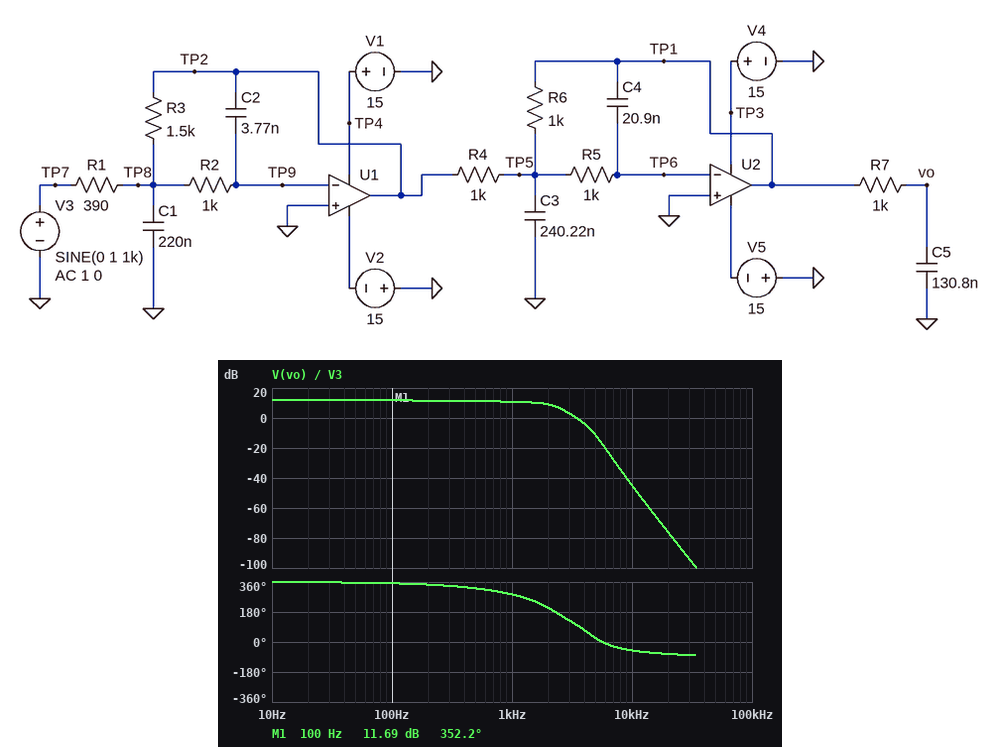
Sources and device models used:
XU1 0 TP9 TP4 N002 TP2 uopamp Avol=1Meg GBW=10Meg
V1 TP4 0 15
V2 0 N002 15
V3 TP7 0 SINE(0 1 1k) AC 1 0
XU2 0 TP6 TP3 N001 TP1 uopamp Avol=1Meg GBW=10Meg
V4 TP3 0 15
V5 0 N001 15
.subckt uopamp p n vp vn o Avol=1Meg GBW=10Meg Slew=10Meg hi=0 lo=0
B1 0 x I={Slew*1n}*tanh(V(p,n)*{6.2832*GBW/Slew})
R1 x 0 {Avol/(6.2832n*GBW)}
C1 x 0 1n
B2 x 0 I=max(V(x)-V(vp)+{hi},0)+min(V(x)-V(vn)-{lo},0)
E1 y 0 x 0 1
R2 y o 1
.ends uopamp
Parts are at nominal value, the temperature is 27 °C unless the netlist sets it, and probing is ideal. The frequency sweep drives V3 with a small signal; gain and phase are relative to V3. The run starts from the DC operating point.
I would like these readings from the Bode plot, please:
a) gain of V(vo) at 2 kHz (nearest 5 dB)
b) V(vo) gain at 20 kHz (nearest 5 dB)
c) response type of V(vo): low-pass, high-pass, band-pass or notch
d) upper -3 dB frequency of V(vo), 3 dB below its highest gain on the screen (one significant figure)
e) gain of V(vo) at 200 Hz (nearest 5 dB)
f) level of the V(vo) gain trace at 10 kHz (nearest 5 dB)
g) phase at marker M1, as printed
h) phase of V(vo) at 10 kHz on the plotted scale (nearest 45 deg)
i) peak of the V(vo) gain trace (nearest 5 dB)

10 dB
-75 dB
low-pass
2 kHz
10 dB
-45 dB
352.2 deg
-45 deg
10 dB
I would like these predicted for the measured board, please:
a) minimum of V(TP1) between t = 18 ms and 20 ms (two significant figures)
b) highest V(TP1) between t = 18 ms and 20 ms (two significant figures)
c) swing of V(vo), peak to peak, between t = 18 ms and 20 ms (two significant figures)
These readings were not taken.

-4.5 V
4.5 V
6.9 V
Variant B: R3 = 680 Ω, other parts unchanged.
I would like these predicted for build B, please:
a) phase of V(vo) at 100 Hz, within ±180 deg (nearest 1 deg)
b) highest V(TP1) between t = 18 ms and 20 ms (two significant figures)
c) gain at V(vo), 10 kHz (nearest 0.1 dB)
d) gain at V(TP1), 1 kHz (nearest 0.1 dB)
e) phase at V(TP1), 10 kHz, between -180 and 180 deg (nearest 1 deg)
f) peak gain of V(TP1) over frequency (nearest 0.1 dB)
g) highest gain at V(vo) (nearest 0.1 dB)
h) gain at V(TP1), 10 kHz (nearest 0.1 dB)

-7 deg
2.0 V
-42.6 dB
6.0 dB
45 deg
7.4 dB
4.8 dB
-24.3 dB
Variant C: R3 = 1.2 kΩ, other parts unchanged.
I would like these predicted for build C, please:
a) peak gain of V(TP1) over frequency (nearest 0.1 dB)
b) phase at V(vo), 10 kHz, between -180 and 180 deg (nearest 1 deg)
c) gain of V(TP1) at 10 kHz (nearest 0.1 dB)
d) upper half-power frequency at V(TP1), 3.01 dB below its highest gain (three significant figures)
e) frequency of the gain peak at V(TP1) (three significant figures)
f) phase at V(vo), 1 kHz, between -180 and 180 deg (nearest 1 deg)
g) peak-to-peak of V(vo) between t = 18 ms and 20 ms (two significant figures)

12.7 dB
-48 deg
-26.0 dB
2.90 kHz
1.90 kHz
-73 deg
5.5 V
